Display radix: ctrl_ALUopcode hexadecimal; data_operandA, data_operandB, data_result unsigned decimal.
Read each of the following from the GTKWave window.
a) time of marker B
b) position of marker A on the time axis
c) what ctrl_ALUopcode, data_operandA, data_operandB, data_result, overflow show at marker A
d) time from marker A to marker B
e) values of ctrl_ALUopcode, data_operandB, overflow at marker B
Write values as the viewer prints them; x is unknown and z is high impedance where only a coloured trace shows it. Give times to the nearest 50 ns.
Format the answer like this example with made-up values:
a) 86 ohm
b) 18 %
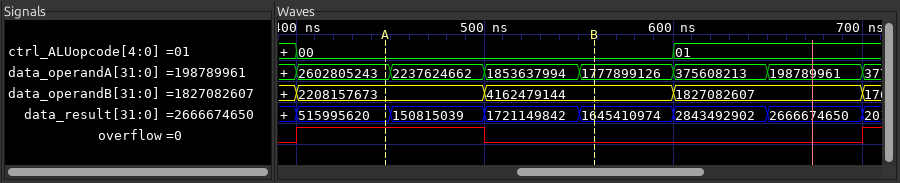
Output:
a) 550 ns
b) 450 ns
c) ctrl_ALUopcode=00, data_operandA=2602805243, data_operandB=2208157673, data_result=515995620, overflow=1
d) 100 ns
e) ctrl_ALUopcode=00, data_operandB=4162479144, overflow=0
